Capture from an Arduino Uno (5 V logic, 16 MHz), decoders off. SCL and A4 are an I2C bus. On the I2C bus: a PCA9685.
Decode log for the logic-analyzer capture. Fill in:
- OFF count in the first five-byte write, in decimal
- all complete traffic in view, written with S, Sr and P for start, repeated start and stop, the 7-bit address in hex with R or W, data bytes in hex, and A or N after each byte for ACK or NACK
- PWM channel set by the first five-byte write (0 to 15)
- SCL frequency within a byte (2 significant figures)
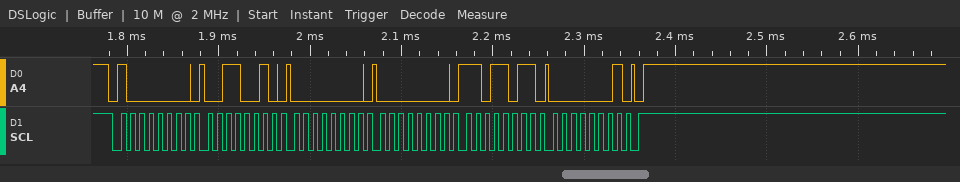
475
S 40W A 32 A 00 A 00 A DB A 01 A P
11
100 kHz
